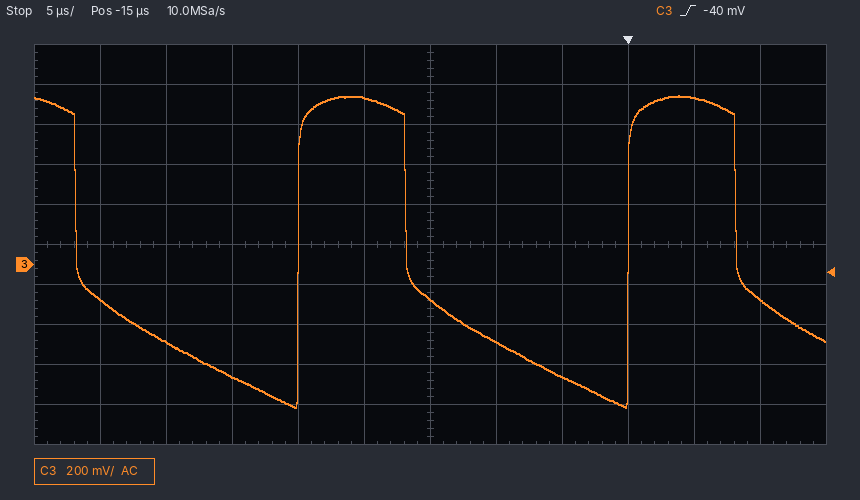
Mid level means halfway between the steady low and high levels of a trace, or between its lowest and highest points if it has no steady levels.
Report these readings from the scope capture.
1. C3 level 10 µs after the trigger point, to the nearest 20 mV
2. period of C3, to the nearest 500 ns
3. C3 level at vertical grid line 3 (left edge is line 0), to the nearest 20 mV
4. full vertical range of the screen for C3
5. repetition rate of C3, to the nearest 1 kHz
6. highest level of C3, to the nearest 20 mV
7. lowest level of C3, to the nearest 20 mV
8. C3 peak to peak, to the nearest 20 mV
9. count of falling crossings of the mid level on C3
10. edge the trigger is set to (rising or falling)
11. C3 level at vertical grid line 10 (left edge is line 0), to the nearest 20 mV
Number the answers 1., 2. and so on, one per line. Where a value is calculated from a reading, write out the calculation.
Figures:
1. -180 mV
2. 25.0 µs
3. -560 mV
4. 2 V
5. 1 / 25.0 µs ≈ 40 kHz
6. 840 mV
7. -720 mV
8. 840 mV − (-720 mV) = 1.56 V
9. 3
10. rising
11. 840 mV
